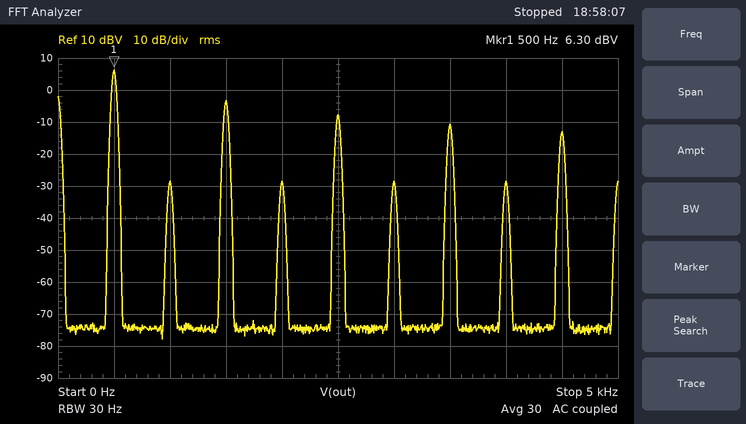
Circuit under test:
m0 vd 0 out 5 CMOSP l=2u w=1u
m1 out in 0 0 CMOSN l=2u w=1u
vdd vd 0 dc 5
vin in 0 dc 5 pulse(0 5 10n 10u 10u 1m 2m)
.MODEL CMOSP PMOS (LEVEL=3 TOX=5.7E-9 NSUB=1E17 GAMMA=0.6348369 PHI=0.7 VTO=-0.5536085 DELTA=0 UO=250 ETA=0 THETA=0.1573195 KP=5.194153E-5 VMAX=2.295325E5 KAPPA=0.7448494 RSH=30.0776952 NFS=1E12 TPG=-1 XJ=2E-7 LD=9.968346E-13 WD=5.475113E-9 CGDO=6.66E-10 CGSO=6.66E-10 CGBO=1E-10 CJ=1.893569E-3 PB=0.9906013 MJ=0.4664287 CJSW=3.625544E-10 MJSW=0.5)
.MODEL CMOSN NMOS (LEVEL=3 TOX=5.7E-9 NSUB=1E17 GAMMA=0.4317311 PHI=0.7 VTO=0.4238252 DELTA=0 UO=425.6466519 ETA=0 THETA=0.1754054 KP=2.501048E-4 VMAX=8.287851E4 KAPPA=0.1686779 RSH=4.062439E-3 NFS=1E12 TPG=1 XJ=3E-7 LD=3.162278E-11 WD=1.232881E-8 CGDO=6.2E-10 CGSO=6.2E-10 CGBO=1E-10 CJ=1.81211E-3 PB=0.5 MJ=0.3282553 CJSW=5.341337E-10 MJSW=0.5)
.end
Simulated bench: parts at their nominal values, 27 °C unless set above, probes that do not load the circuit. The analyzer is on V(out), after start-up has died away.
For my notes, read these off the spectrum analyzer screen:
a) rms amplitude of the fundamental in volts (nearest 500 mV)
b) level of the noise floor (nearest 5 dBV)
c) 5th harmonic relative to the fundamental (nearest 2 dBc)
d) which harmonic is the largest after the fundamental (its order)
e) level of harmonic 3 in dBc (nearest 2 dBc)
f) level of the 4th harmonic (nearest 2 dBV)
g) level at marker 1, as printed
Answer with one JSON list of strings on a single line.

["2.0 V", "-75 dBV", "-14 dBc", "3", "-10 dBc", "-28 dBV", "6.30 dBV"]
